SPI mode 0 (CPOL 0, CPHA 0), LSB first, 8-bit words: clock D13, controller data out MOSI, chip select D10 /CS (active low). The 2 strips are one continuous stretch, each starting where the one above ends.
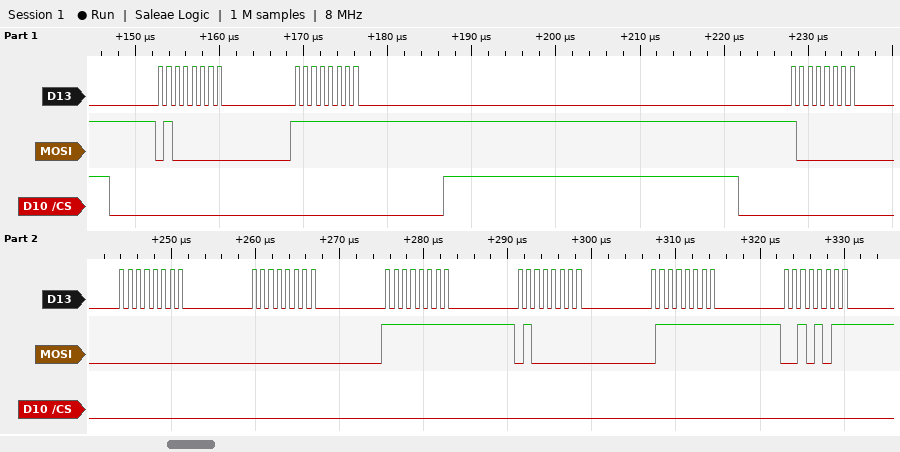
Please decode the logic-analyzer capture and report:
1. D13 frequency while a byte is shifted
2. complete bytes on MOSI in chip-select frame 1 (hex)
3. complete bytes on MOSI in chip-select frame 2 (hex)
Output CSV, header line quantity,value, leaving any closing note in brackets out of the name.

quantity,value
D13 frequency while a byte is shifted,1 MHz
complete bytes on MOSI in chip-select frame 1,02 FF
complete bytes on MOSI in chip-select frame 2,01 00 00 FF 02 FE D4
